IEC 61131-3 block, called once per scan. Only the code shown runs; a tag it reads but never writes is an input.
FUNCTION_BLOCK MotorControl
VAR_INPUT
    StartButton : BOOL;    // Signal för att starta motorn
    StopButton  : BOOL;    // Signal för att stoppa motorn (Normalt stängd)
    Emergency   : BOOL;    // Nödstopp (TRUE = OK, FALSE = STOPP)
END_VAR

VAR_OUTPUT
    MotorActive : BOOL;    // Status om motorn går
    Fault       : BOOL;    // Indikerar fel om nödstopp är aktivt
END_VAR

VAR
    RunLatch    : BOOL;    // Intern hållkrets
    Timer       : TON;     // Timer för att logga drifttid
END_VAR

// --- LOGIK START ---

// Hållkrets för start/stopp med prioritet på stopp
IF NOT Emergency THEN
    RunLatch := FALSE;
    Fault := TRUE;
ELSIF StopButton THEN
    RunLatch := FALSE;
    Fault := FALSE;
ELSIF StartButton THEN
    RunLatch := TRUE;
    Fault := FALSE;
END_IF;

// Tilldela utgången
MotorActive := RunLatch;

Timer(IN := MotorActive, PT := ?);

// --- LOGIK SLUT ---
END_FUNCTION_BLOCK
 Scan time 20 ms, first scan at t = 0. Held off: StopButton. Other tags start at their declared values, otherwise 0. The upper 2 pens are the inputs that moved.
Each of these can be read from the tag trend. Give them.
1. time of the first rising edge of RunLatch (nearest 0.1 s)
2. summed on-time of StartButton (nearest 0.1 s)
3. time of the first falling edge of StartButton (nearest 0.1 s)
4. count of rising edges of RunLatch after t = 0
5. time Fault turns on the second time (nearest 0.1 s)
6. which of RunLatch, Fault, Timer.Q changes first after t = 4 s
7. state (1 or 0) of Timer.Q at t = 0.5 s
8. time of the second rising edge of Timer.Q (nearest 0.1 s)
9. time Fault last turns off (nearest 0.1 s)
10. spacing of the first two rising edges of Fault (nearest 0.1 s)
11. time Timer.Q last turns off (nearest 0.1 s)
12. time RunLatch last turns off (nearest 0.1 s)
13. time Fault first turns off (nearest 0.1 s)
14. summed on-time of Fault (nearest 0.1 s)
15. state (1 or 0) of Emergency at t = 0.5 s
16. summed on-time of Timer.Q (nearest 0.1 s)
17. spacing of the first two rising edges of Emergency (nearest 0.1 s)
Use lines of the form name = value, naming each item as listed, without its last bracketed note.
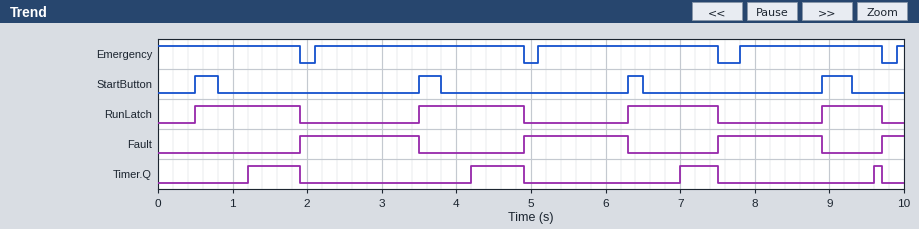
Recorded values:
time of the first rising edge of RunLatch = 0.5 s
summed on-time of StartButton = 1.2 s
time of the first falling edge of StartButton = 0.8 s
count of rising edges of RunLatch after t = 0 = 4
time Fault turns on the second time = 4.9 s
which of RunLatch, Fault, Timer.Q changes first after t = 4 s = Timer.Q
state (1 or 0) of Timer.Q at t = 0.5 s = 0
time of the second rising edge of Timer.Q = 4.2 s
time Fault last turns off = 8.9 s
spacing of the first two rising edges of Fault = 3.0 s
time Timer.Q last turns off = 9.7 s
time RunLatch last turns off = 9.7 s
time Fault first turns off = 3.5 s
summed on-time of Fault = 4.7 s
state (1 or 0) of Emergency at t = 0.5 s = 1
summed on-time of Timer.Q = 2.0 s
spacing of the first two rising edges of Emergency = 3.0 s
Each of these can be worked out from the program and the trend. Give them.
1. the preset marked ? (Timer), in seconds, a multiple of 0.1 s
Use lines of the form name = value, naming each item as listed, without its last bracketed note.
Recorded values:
the preset marked ? (Timer), in seconds, a multiple of 0.1 s = 0.7 s
